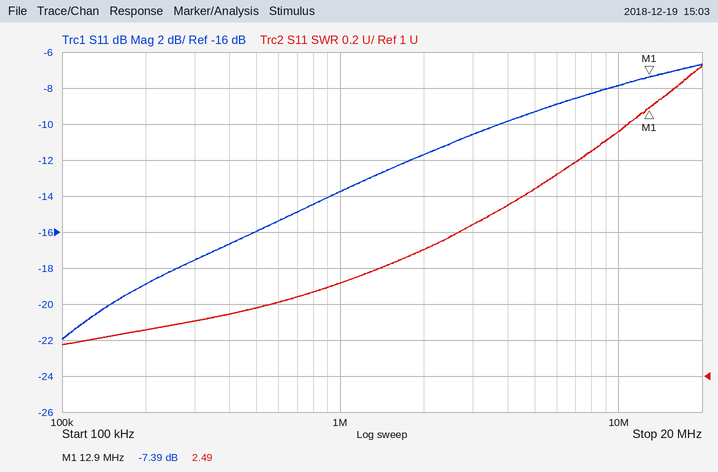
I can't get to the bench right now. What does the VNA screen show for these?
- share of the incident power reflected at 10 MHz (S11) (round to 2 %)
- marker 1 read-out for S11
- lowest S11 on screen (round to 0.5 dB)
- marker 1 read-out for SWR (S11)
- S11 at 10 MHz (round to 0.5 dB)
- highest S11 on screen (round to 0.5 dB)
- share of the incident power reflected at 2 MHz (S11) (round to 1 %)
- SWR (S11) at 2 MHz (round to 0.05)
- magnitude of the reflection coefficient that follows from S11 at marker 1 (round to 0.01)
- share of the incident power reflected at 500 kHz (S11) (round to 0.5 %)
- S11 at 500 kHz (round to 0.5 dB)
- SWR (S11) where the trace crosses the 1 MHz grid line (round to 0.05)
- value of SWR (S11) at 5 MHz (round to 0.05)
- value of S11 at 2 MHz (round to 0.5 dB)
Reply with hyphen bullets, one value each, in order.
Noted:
- 16 %
- -7.39 dB
- -22.0 dB
- 2.49
- -8.0 dB
- -6.5 dB
- 7 %
- 1.70
- 0.43
- 2.5 %
- -16.0 dB
- 1.50
- 2.05
- -11.5 dB
